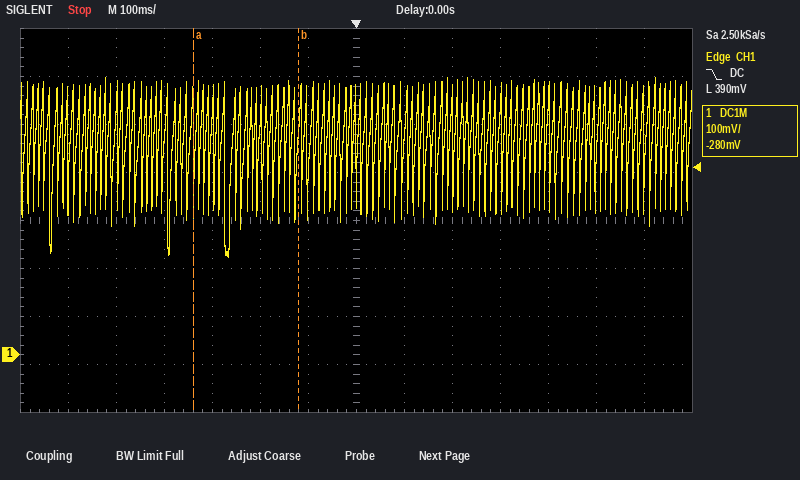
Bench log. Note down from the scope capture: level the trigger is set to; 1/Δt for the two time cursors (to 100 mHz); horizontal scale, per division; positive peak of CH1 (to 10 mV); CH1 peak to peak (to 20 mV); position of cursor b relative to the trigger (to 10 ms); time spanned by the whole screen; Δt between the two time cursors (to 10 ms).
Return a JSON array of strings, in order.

["390 mV", "4.5 Hz", "100 ms", "580 mV", "380 mV", "-120 ms", "1.4 s", "220 ms"]
